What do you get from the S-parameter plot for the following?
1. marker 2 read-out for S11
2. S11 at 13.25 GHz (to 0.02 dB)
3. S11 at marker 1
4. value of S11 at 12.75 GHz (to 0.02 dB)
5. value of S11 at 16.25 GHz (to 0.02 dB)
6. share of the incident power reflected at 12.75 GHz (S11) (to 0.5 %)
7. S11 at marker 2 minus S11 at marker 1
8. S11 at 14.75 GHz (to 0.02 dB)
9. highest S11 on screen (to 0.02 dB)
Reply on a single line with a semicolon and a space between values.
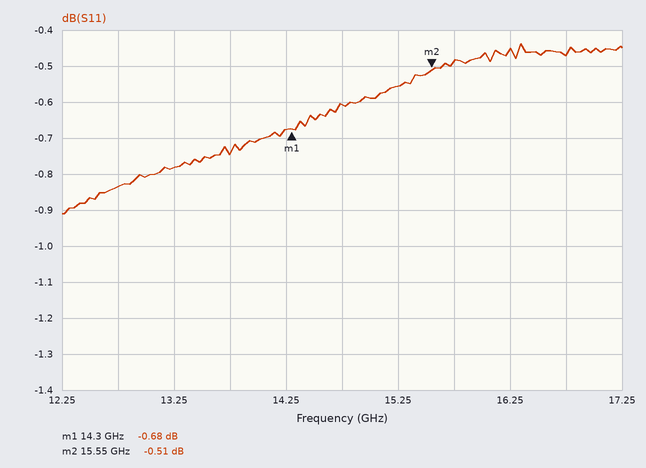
-0.51 dB; -0.78 dB; -0.68 dB; -0.84 dB; -0.46 dB; 82.5 %; 0.17 dB; -0.60 dB; -0.44 dB
